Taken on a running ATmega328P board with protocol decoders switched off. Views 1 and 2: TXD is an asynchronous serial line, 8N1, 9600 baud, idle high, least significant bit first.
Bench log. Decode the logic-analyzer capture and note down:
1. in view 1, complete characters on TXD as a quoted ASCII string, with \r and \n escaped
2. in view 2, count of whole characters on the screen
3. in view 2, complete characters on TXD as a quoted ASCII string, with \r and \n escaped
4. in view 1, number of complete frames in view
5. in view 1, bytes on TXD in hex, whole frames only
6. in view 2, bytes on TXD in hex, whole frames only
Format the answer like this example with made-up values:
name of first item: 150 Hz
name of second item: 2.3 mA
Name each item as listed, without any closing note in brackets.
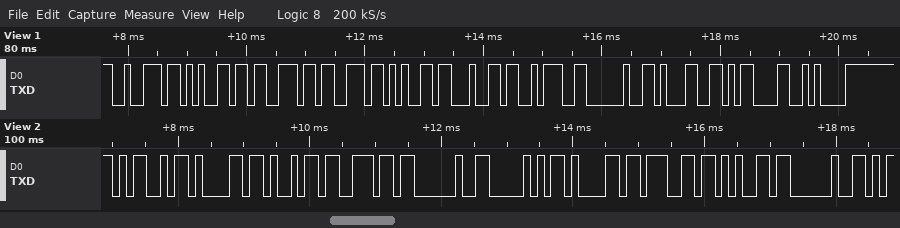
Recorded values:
in view 1, complete characters on TXD as a quoted ASCII string, with \r and \n escaped: "ressed: 1\r\n"
in view 2, count of whole characters on the screen: 10
in view 2, complete characters on TXD as a quoted ASCII string, with \r and \n escaped: "Main Page "
in view 1, number of complete frames in view: 11
in view 1, bytes on TXD in hex, whole frames only: 0x72 0x65 0x73 0x73 0x65 0x64 0x3A 0x20 0x31 0x0D 0x0A
in view 2, bytes on TXD in hex, whole frames only: 4D 61 69 6E 20 50 61 67 65 20
